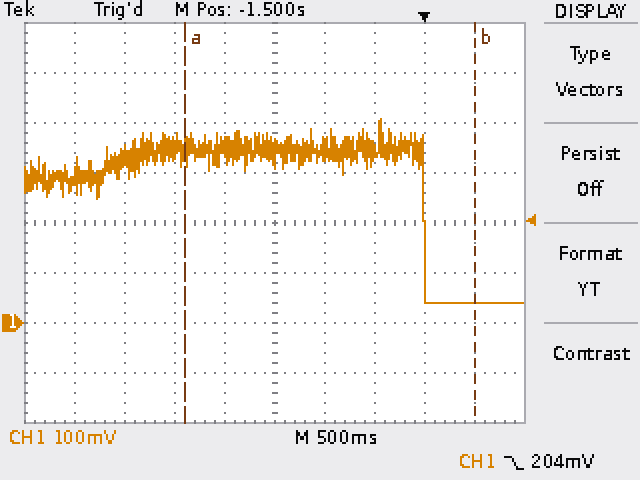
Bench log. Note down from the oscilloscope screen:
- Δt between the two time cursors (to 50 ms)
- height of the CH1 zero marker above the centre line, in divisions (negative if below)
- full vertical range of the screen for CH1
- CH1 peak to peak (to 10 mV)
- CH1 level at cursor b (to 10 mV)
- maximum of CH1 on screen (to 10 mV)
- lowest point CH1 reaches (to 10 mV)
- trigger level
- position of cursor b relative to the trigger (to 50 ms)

2.90 s
-2.0 div
800 mV
370 mV
40 mV
410 mV
40 mV
204 mV
+500 ms
